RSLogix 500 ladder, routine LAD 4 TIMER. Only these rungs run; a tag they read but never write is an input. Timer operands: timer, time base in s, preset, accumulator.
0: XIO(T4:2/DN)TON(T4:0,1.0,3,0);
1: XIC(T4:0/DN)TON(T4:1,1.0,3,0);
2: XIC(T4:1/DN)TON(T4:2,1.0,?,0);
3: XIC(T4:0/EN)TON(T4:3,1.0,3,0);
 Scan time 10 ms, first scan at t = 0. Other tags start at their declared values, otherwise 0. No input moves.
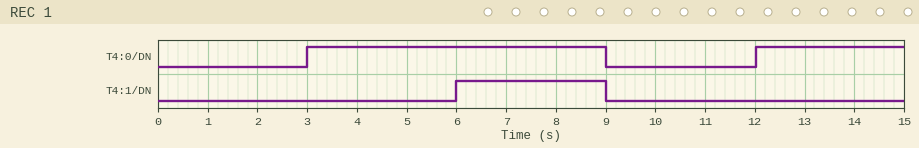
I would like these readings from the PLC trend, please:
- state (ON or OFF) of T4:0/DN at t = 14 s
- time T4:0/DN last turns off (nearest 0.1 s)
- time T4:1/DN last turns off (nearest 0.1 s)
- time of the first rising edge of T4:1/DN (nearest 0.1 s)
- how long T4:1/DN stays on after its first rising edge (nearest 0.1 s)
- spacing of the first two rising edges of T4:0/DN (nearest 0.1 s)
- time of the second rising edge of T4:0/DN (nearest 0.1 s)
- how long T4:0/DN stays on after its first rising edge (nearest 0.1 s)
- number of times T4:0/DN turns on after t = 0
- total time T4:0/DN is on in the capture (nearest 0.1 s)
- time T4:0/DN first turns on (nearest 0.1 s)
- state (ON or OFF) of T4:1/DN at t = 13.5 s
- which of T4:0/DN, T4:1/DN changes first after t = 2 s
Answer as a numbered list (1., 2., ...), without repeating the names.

1. ON
2. 9.0 s
3. 9.0 s
4. 6.0 s
5. 3.0 s
6. 9.0 s
7. 12.0 s
8. 6.0 s
9. 2
10. 9.0 s
11. 3.0 s
12. OFF
13. T4:0/DN
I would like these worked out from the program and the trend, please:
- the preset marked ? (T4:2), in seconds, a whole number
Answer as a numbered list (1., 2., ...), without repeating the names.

1. 3 s
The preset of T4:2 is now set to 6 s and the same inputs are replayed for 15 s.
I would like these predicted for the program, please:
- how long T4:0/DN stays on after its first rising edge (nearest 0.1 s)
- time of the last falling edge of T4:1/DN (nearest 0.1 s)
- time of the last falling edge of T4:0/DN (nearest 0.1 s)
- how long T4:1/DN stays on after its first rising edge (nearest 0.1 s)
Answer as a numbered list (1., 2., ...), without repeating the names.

1. 9.0 s
2. 12.0 s
3. 12.0 s
4. 6.0 s
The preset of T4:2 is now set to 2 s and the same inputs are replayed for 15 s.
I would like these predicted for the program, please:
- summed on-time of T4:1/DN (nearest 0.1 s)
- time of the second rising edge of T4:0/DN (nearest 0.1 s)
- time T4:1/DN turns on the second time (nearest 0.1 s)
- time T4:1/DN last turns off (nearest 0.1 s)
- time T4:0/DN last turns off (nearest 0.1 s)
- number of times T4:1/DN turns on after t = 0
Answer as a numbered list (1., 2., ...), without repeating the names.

1. 3.0 s
2. 11.0 s
3. 14.0 s
4. 8.0 s
5. 8.0 s
6. 2
